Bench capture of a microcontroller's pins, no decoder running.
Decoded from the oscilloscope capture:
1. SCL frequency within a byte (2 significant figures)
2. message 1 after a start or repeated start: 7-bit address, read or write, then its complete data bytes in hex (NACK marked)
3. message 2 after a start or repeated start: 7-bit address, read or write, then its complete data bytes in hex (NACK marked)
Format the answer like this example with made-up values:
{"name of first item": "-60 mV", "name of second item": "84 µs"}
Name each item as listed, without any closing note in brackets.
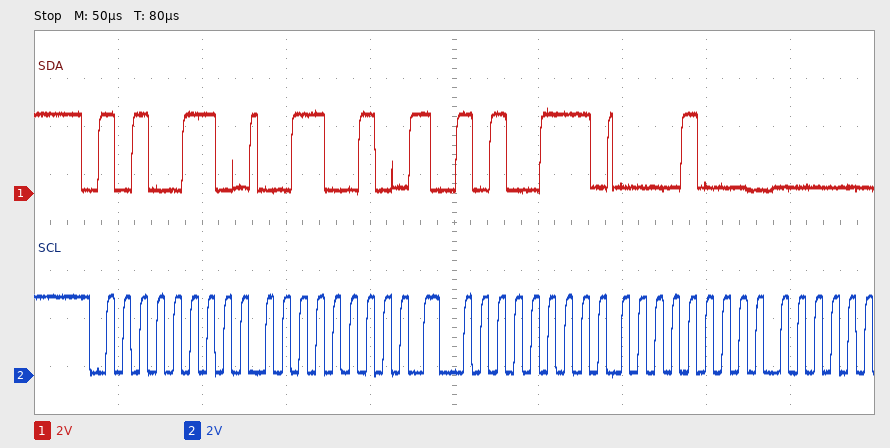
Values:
{"SCL frequency within a byte": "100 kHz", "message 1 after a start or repeated start: 7-bit address, read or write, then its complete data bytes in hex": "0x53 write: 32", "message 2 after a start or repeated start: 7-bit address, read or write, then its complete data bytes in hex": "0x53 read: 08"}
